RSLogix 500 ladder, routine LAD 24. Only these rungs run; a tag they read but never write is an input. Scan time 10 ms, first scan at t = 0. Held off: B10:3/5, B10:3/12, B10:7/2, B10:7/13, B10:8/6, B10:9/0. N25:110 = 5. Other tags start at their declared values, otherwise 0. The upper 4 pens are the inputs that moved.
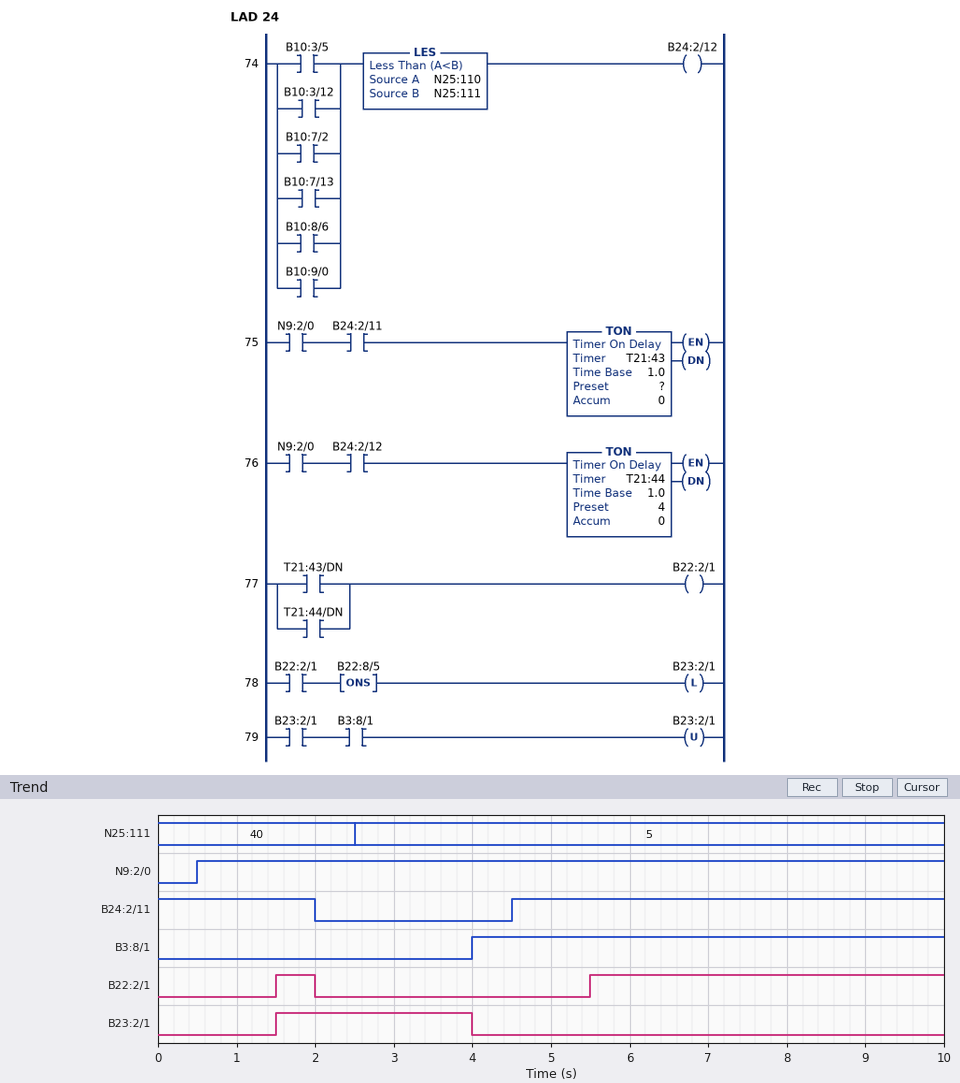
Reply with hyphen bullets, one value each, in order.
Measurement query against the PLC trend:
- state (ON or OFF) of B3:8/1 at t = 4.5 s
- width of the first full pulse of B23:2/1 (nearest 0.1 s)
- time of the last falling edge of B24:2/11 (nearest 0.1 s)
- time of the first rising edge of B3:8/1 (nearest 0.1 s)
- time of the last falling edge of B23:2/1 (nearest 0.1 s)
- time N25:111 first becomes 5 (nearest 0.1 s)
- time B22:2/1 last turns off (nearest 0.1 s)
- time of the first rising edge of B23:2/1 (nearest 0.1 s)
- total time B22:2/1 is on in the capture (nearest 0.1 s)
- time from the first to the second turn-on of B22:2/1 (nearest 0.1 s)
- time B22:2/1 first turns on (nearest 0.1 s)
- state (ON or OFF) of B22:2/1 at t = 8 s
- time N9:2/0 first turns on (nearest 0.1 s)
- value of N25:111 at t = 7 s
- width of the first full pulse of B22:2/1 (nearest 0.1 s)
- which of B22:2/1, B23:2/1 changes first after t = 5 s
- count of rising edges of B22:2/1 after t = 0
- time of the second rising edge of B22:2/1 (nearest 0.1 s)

- ON
- 2.5 s
- 2.0 s
- 4.0 s
- 4.0 s
- 2.5 s
- 2.0 s
- 1.5 s
- 5.0 s
- 4.0 s
- 1.5 s
- ON
- 0.5 s
- 5
- 0.5 s
- B22:2/1
- 2
- 5.5 s
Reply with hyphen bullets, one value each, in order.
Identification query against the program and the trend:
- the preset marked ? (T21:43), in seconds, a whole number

- 1 s
